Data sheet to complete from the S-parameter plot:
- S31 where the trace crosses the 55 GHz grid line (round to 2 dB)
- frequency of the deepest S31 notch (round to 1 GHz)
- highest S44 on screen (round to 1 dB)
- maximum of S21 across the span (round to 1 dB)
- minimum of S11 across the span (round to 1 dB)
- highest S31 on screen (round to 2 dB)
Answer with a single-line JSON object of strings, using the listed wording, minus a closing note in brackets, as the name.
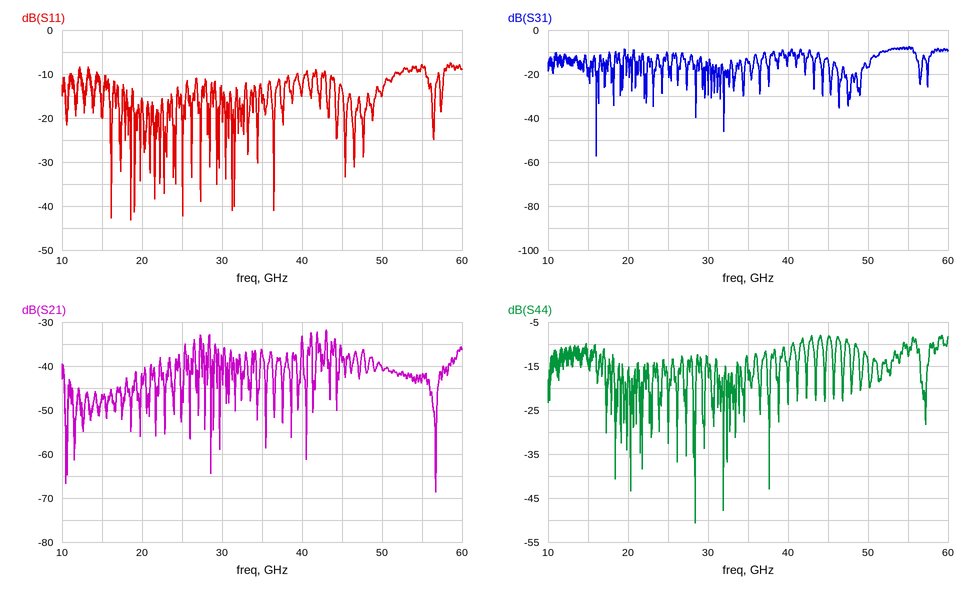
{"S31 where the trace crosses the 55 GHz grid line": "-8 dB", "frequency of the deepest S31 notch": "16 GHz", "highest S44 on screen": "-8 dB", "maximum of S21 across the span": "-32 dB", "minimum of S11 across the span": "-43 dB", "highest S31 on screen": "-8 dB"}
